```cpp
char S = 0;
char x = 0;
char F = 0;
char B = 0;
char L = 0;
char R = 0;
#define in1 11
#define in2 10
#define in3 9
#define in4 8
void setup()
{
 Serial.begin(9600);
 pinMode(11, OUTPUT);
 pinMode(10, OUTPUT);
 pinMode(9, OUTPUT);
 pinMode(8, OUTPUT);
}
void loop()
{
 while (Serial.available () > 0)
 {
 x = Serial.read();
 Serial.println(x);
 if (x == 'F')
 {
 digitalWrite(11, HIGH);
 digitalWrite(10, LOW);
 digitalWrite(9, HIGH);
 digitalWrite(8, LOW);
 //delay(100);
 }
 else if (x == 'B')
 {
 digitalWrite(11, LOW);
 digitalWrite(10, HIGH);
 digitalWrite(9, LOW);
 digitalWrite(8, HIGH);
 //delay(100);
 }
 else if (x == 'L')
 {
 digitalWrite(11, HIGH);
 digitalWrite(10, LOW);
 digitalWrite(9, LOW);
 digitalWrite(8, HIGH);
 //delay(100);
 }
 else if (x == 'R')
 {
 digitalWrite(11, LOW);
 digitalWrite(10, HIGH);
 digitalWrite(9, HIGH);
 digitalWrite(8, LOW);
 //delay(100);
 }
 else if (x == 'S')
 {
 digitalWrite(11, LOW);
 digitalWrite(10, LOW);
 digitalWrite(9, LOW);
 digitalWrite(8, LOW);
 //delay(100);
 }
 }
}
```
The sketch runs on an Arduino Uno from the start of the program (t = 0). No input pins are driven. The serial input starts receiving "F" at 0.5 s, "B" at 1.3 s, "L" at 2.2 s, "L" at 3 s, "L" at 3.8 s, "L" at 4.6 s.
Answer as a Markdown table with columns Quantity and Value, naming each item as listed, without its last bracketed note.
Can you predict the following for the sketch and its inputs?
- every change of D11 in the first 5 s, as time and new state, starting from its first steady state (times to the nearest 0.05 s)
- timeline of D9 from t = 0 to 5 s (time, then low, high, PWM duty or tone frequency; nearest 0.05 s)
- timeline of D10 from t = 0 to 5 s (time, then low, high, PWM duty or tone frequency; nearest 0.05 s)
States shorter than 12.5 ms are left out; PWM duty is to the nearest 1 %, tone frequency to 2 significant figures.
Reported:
| Quantity | Value |
|---|---|
| every change of D11 in the first 5 s, as time and new state, starting from its first steady state | 0 s low; 0.5 s high; 1.3 s low; 2.2 s high |
| timeline of D9 from t = 0 to 5 s | 0 s low; 0.5 s high; 1.3 s low |
| timeline of D10 from t = 0 to 5 s | 0 s low; 1.3 s high; 2.2 s low |
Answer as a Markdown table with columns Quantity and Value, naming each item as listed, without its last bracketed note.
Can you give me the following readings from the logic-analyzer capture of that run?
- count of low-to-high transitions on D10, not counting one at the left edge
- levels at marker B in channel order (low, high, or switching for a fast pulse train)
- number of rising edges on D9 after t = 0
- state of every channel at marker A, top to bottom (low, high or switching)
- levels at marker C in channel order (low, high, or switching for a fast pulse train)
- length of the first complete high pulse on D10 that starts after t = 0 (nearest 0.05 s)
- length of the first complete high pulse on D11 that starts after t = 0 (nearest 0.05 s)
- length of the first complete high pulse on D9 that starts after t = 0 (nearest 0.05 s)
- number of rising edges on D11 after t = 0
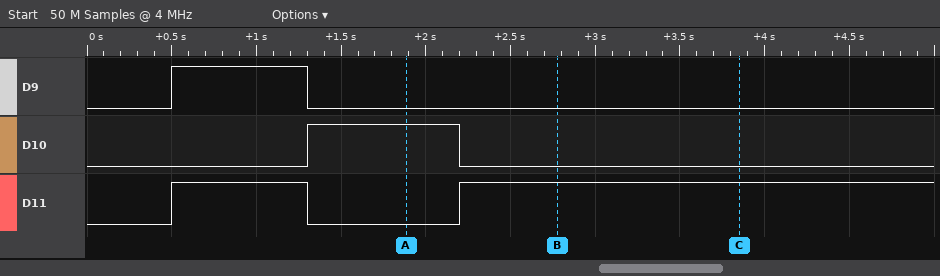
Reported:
| Quantity | Value |
|---|---|
| count of low-to-high transitions on D10, not counting one at the left edge | 1 |
| levels at marker B in channel order | D9 low, D10 low, D11 high |
| number of rising edges on D9 after t = 0 | 1 |
| state of every channel at marker A, top to bottom | D9 low, D10 high, D11 low |
| levels at marker C in channel order | D9 low, D10 low, D11 high |
| length of the first complete high pulse on D10 that starts after t = 0 | 0.90 s |
| length of the first complete high pulse on D11 that starts after t = 0 | 0.80 s |
| length of the first complete high pulse on D9 that starts after t = 0 | 0.80 s |
| number of rising edges on D11 after t = 0 | 2 |
